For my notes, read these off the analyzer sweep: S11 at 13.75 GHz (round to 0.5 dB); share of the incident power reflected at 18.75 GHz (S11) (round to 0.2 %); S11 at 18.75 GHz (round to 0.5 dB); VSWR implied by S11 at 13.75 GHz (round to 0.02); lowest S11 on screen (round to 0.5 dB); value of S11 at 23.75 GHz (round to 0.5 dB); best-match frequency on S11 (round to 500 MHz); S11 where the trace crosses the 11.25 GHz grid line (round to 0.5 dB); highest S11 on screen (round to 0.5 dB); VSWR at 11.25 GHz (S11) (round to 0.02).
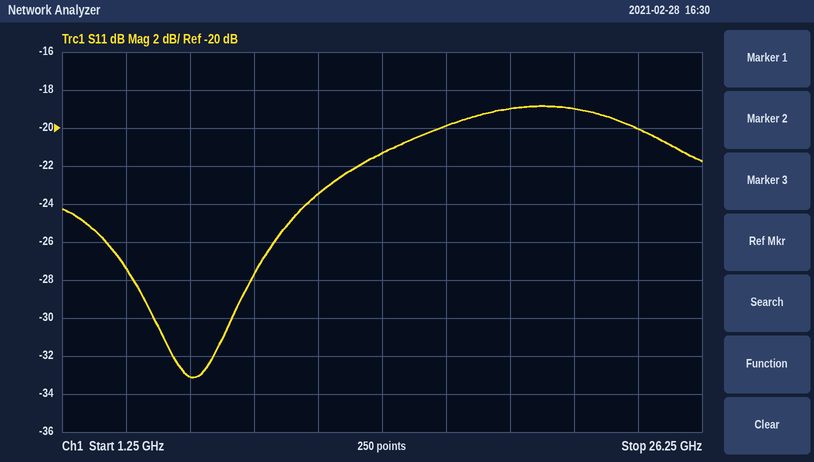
-21.5 dB
1.2 %
-19.0 dB
1.18
-33.0 dB
-20.0 dB
6.5 GHz
-23.5 dB
-19.0 dB
1.14
